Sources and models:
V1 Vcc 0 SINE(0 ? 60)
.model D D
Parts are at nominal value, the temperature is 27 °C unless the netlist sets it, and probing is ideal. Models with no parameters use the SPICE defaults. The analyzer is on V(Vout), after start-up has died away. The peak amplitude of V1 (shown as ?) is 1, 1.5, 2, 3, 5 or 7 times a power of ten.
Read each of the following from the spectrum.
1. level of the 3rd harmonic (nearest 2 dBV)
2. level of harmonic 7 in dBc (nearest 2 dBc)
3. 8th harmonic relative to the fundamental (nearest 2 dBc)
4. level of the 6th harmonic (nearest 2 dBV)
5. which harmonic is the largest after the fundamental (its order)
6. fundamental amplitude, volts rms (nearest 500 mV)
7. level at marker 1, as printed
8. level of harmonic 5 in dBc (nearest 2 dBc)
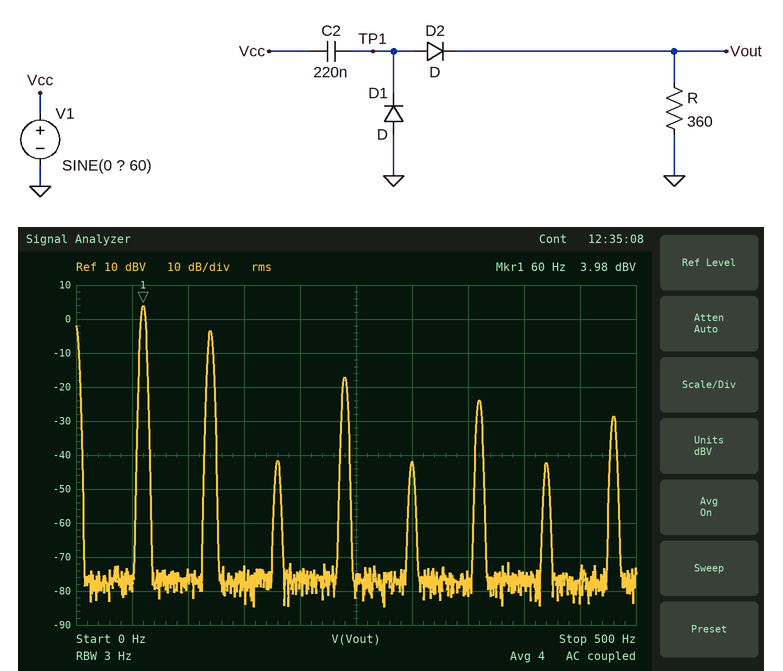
-42 dBV
-46 dBc
-32 dBc
-24 dBV
2
1.5 V
3.98 dBV
-46 dBc
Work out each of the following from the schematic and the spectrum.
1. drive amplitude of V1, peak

150 V
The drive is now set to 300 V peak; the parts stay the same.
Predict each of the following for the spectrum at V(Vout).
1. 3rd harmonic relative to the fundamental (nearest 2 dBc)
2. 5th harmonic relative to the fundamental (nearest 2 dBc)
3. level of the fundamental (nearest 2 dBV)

-52 dBc
-52 dBc
10 dBV
